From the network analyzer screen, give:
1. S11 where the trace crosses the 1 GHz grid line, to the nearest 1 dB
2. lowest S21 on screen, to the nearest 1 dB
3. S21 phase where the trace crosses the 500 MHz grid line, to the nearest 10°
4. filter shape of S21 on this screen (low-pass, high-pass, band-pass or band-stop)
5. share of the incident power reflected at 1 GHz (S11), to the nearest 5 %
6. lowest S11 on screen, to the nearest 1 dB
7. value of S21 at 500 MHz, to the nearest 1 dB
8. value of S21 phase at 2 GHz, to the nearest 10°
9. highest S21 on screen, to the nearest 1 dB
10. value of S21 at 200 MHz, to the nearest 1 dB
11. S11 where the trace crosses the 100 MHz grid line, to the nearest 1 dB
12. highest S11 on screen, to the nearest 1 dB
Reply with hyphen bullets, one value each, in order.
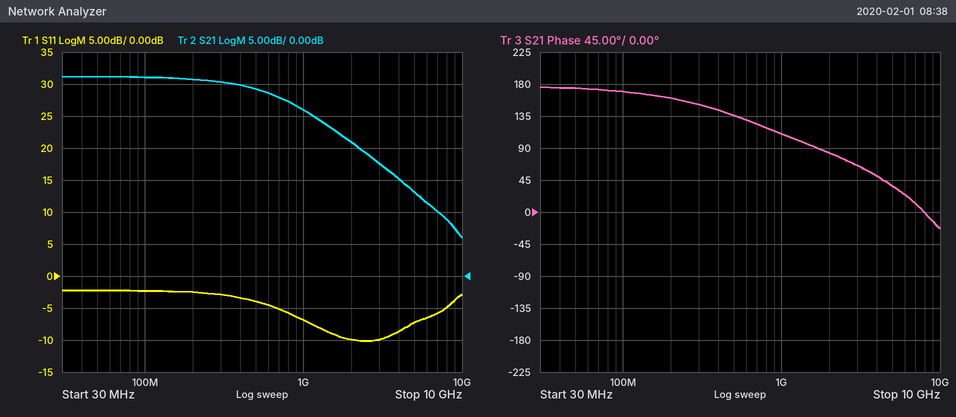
- -7 dB
- 6 dB
- 140°
- low-pass
- 20 %
- -10 dB
- 29 dB
- 80°
- 31 dB
- 31 dB
- -2 dB
- -2 dB
